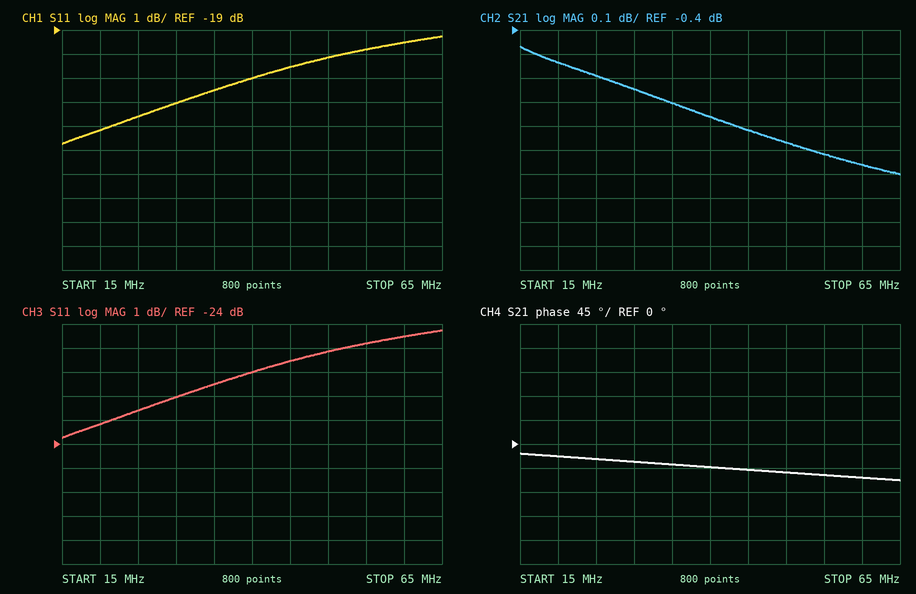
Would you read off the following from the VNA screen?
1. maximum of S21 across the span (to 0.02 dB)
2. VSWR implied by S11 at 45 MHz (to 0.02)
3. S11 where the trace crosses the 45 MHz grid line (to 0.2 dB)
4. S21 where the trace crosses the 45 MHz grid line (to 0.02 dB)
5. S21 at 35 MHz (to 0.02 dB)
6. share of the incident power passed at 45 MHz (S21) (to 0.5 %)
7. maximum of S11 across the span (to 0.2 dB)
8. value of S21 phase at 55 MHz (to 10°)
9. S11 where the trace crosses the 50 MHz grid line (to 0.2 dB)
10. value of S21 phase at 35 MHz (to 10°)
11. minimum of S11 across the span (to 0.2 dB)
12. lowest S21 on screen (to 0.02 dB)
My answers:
-0.46 dB
1.20
-20.6 dB
-0.82 dB
-0.70 dB
83.0 %
-19.2 dB
-60°
-20.2 dB
-40°
-23.8 dB
-1.00 dB
